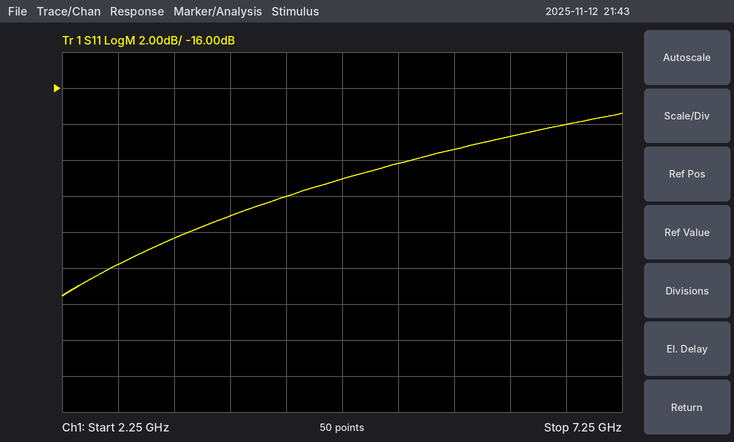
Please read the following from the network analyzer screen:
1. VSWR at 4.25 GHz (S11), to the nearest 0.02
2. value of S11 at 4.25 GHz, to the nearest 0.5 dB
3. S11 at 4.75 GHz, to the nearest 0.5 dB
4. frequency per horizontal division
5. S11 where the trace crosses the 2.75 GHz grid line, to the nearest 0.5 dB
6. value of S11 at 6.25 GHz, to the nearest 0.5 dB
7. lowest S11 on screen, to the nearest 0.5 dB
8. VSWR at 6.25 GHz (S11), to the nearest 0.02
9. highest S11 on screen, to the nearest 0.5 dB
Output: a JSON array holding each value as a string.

["1.18", "-22.0 dB", "-21.0 dB", "500 MHz", "-26.0 dB", "-18.5 dB", "-27.5 dB", "1.26", "-17.5 dB"]
